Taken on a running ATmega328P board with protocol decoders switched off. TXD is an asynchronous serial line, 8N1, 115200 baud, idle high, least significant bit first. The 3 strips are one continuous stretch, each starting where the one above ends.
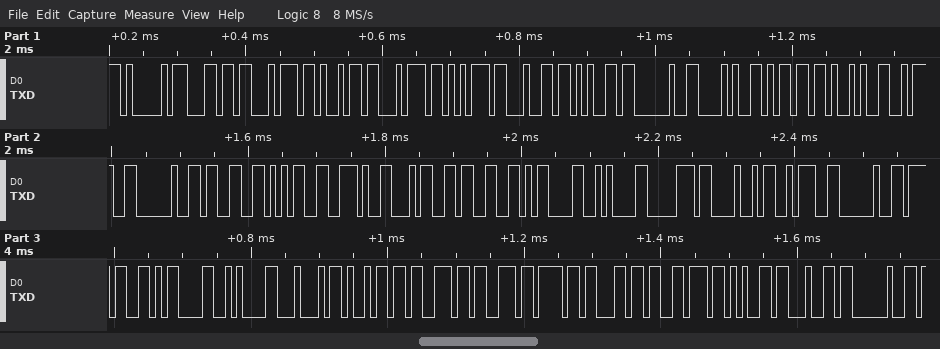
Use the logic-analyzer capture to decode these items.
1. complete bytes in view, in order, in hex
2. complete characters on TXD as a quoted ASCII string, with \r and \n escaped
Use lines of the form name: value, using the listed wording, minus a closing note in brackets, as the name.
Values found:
complete bytes in view, in order, in hex: 41 6C 74 69 74 75 64 65 20 28 6D 29 3A 20 33 35 2E 34 33 0D 0A 70 48 3A 20 37 0D 0A 44 69 73 73 6F 6C 76 65 64 20
complete characters on TXD as a quoted ASCII string, with \r and \n escaped: "Altitude (m): 35.43\r\npH: 7\r\nDissolved "
